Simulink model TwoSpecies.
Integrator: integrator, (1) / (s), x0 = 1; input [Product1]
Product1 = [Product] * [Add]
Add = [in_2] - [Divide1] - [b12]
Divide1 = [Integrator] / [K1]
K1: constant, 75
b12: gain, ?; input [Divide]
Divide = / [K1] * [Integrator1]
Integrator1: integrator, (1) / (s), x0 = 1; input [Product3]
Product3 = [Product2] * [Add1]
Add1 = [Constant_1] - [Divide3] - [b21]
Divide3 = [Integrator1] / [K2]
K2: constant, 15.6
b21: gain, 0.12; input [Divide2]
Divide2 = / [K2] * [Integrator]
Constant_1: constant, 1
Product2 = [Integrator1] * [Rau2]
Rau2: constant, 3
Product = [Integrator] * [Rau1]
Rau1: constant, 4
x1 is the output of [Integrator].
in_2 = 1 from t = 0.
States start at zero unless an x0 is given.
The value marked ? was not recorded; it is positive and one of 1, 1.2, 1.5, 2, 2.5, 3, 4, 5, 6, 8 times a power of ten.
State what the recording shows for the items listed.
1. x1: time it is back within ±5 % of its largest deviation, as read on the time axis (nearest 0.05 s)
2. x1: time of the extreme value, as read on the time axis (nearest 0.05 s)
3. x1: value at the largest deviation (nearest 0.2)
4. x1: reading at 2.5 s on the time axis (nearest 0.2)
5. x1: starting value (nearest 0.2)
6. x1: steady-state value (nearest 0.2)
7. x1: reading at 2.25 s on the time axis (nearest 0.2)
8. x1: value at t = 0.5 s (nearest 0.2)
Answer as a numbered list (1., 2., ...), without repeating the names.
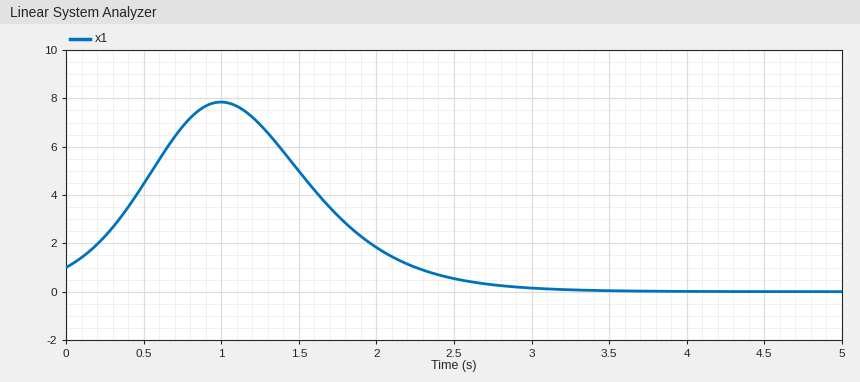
1. 2.70 s
2. 1.00 s
3. 7.8
4. 0.6
5. 1.0
6. 0.0
7. 1.0
8. 4.4
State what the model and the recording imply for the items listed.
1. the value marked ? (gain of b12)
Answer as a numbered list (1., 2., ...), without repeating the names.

1. 8
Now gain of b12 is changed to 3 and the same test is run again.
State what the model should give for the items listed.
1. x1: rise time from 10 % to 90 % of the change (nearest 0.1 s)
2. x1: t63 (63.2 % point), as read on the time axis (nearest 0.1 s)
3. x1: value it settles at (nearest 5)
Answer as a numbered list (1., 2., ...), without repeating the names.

1. 1.7 s
2. 1.3 s
3. 45
